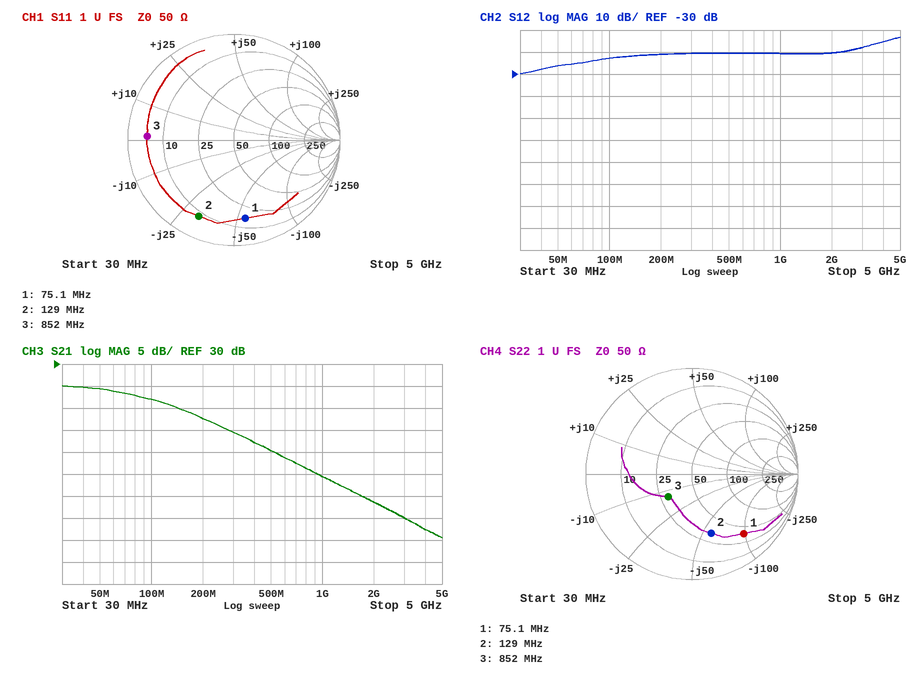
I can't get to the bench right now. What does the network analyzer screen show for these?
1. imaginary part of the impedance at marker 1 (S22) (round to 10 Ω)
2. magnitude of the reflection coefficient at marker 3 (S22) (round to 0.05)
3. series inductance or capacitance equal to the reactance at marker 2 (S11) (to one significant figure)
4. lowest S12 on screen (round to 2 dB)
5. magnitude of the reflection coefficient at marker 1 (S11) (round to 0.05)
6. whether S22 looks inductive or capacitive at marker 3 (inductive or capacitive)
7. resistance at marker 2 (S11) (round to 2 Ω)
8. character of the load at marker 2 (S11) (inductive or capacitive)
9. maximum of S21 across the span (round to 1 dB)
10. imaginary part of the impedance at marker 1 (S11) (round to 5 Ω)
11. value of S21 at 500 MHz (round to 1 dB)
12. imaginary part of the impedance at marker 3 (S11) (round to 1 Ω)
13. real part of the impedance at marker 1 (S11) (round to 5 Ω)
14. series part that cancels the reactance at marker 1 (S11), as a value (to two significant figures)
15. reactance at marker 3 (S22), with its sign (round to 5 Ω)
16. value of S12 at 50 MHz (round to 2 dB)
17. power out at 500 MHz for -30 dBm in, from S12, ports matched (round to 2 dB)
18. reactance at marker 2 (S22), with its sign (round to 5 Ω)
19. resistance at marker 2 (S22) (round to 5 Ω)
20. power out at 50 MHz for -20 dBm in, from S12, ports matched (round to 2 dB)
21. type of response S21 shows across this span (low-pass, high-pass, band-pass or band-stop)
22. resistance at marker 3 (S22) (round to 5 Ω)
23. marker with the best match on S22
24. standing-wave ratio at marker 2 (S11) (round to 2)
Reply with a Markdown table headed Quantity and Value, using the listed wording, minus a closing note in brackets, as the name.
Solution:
| Quantity | Value |
|---|---|
| imaginary part of the impedance at marker 1 (S22) | -100 Ω |
| magnitude of the reflection coefficient at marker 3 (S22) | 0.30 |
| series inductance or capacitance equal to the reactance at marker 2 (S11) | 40 pF |
| lowest S12 on screen | -30 dB |
| magnitude of the reflection coefficient at marker 1 (S11) | 0.75 |
| whether S22 looks inductive or capacitive at marker 3 | capacitive |
| resistance at marker 2 (S11) | 8 Ω |
| character of the load at marker 2 (S11) | capacitive |
| maximum of S21 across the span | 25 dB |
| imaginary part of the impedance at marker 1 (S11) | -55 Ω |
| value of S21 at 500 MHz | 10 dB |
| imaginary part of the impedance at marker 3 (S11) | +1 Ω |
| real part of the impedance at marker 1 (S11) | 15 Ω |
| series part that cancels the reactance at marker 1 (S11), as a value | 120 nH |
| reactance at marker 3 (S22), with its sign | -15 Ω |
| value of S12 at 50 MHz | -26 dB |
| power out at 500 MHz for -30 dBm in, from S12, ports matched | -50 dBm |
| reactance at marker 2 (S22), with its sign | -55 Ω |
| resistance at marker 2 (S22) | 35 Ω |
| power out at 50 MHz for -20 dBm in, from S12, ports matched | -46 dBm |
| type of response S21 shows across this span | low-pass |
| resistance at marker 3 (S22) | 30 Ω |
| marker with the best match on S22 | marker 3 |
| standing-wave ratio at marker 2 (S11) | 8 |
